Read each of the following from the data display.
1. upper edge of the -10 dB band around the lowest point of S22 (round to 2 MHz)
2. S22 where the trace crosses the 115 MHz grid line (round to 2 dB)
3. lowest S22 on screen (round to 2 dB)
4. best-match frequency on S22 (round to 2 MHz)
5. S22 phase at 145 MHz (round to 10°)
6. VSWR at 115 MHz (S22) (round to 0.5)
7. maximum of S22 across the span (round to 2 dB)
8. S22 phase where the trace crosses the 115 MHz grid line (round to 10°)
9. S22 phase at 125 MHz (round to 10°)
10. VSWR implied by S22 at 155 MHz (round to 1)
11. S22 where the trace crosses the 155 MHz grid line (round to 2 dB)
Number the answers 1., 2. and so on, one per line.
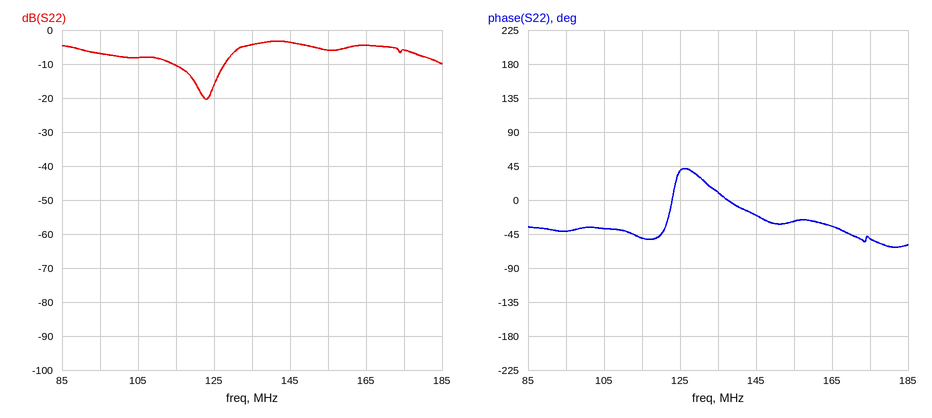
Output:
1. 128 MHz
2. -10 dB
3. -20 dB
4. 122 MHz
5. -20°
6. 2.0
7. -4 dB
8. -50°
9. 40°
10. 3
11. -6 dB
